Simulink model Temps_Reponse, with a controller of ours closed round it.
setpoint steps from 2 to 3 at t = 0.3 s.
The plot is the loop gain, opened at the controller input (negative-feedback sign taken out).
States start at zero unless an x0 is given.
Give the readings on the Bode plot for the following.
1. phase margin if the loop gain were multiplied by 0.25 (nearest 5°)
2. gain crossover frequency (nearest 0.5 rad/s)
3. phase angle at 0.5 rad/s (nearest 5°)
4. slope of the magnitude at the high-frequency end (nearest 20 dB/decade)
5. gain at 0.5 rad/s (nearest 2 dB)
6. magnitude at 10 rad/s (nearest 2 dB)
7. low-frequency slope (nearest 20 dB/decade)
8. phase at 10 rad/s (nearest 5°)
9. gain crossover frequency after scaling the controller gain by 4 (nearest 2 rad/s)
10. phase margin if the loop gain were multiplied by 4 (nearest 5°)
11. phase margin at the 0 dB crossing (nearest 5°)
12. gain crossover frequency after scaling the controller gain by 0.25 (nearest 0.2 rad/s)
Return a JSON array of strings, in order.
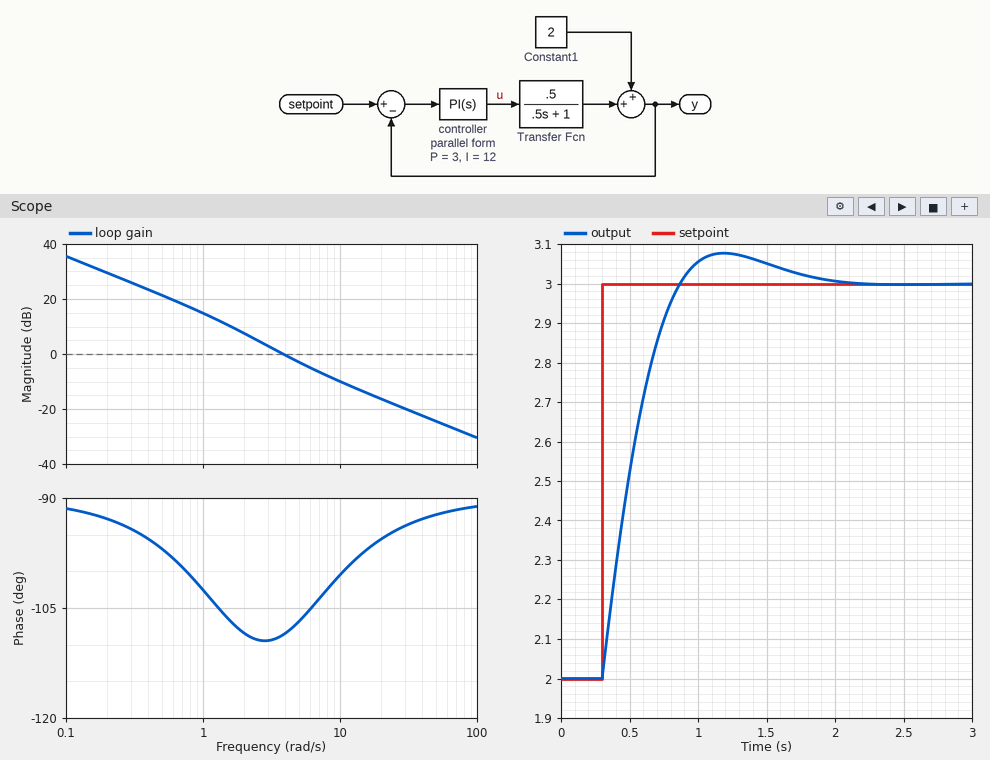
["75°", "4.0 rad/s", "-95°", "-20 dB/decade", "22 dB", "-10 dB", "-20 dB/decade", "-100°", "12 rad/s", "80°", "70°", "1.4 rad/s"]
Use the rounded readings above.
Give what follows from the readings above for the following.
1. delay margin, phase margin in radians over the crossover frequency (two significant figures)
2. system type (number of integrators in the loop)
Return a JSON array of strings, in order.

["0.31 s", "1"]
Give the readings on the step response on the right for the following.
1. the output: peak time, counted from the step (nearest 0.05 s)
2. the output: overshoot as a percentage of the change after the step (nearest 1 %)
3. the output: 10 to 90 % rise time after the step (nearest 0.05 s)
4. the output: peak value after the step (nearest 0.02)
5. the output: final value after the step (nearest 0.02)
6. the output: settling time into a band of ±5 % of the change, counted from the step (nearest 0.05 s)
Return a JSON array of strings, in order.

["0.90 s", "8 %", "0.40 s", "3.08", "3.00", "1.20 s"]
